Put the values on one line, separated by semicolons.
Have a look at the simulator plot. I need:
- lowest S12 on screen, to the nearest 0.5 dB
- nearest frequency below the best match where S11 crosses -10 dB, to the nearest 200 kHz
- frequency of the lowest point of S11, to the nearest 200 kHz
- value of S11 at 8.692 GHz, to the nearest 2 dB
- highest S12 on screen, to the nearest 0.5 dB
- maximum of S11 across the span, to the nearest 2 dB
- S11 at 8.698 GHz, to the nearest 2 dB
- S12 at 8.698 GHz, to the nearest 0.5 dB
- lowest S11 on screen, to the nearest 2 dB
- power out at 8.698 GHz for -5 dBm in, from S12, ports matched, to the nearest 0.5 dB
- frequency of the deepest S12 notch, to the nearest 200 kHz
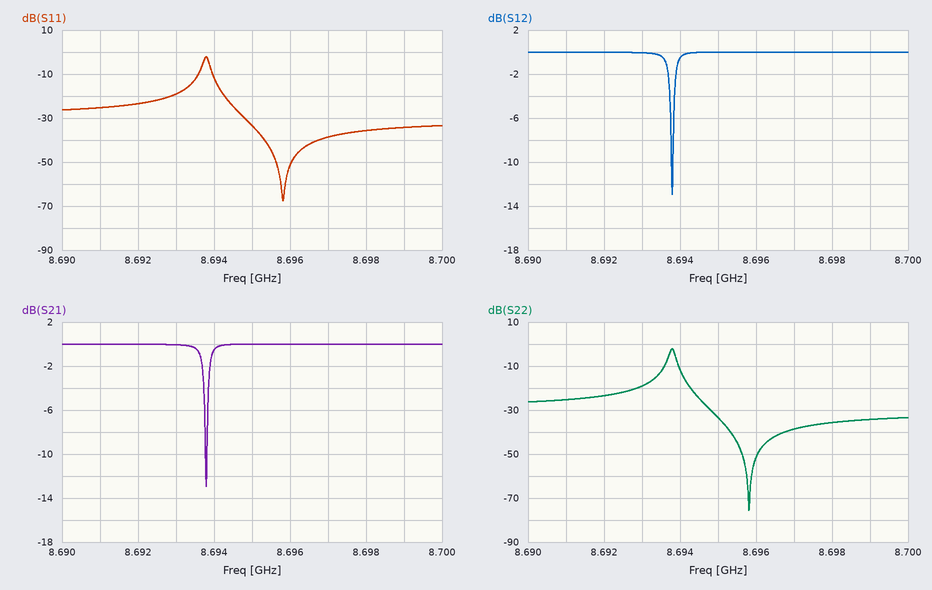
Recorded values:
-13.0 dB; 8.6940 GHz; 8.6958 GHz; -24 dB; 0.0 dB; -2 dB; -36 dB; 0.0 dB; -68 dB; -5.0 dBm; 8.6938 GHz
